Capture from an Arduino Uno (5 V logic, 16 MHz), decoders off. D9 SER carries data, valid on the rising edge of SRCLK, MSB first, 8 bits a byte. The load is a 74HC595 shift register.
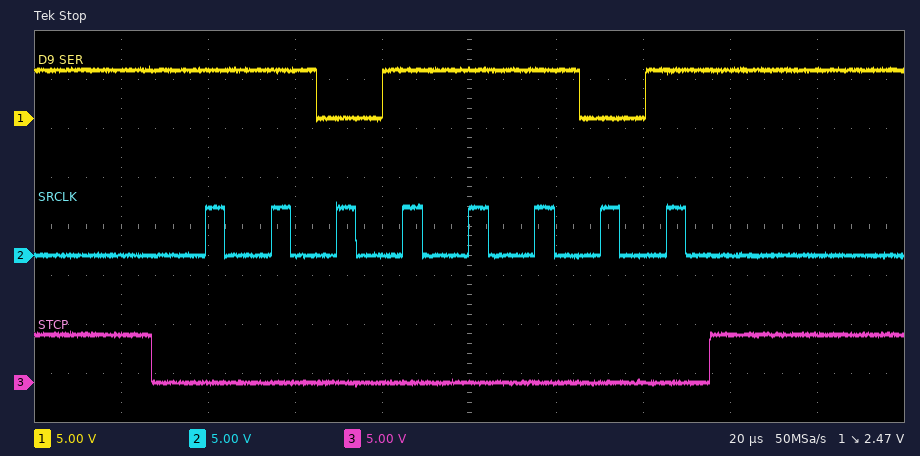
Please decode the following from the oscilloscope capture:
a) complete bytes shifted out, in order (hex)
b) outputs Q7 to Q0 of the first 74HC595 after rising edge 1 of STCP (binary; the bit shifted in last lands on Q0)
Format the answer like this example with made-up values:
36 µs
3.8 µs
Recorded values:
DD
11011101
